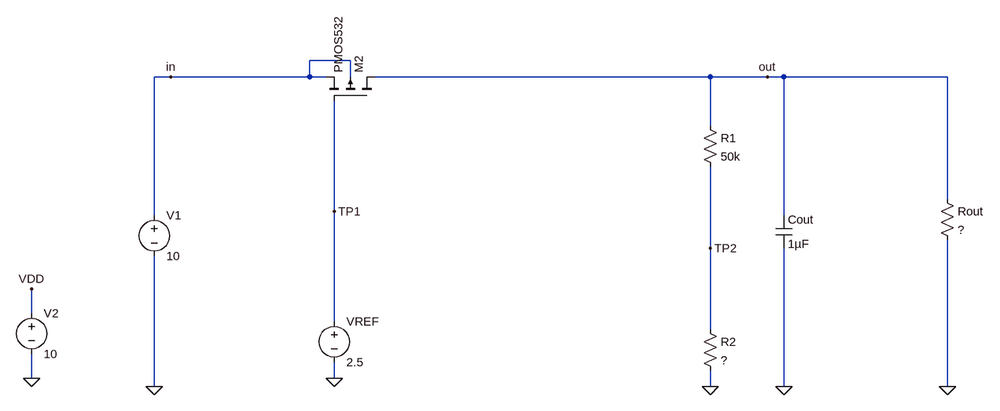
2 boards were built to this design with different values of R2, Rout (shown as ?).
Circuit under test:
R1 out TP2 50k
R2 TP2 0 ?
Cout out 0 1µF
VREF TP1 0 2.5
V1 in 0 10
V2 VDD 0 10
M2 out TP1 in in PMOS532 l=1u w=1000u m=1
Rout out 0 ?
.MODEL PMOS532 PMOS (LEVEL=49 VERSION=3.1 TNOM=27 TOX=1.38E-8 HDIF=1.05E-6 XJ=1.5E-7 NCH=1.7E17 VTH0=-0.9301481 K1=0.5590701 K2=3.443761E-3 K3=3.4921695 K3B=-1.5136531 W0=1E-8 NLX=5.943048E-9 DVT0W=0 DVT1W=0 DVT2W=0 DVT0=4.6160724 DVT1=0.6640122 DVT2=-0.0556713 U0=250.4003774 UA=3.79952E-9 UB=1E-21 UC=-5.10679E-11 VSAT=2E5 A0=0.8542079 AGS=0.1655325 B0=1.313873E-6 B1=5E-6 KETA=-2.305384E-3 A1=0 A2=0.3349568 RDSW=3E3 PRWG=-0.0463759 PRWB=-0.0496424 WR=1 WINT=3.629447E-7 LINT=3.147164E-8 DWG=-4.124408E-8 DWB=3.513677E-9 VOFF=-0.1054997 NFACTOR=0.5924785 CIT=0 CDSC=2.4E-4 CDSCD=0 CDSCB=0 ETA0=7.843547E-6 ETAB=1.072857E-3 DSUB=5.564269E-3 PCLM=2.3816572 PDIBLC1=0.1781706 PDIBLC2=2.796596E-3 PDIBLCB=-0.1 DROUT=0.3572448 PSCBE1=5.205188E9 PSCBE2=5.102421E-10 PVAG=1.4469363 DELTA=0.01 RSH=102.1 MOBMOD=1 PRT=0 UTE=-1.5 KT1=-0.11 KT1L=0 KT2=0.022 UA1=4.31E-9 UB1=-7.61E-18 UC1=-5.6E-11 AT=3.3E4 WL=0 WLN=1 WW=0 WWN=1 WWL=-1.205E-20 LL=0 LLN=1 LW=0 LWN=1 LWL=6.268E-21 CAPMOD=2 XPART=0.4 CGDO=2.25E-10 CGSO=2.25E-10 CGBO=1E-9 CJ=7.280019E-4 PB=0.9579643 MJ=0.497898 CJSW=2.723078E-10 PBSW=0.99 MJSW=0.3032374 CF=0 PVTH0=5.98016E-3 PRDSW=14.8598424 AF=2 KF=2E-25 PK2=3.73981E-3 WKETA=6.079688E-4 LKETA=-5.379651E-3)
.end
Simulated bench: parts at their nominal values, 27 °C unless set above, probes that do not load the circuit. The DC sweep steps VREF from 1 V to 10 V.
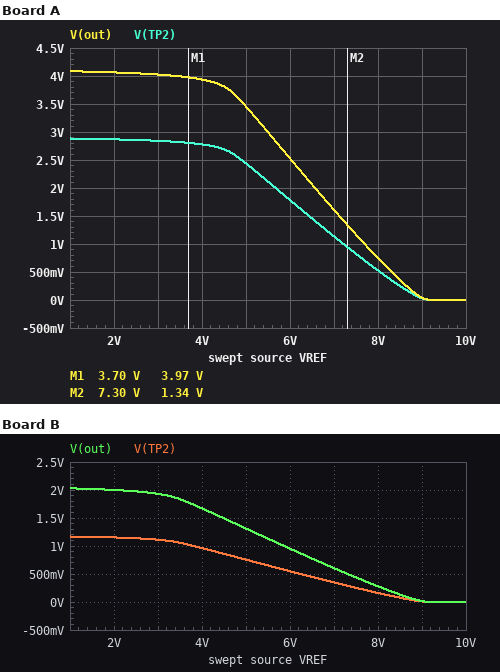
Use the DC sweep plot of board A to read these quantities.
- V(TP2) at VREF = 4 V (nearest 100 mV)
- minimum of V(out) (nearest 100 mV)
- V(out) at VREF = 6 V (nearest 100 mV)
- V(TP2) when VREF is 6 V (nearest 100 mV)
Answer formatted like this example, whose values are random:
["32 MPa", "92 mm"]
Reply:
["2.8 V", "0 V", "2.5 V", "1.8 V"]
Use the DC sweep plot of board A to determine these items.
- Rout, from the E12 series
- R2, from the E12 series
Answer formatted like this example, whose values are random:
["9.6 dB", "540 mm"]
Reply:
["150 Ω", "120 kΩ"]
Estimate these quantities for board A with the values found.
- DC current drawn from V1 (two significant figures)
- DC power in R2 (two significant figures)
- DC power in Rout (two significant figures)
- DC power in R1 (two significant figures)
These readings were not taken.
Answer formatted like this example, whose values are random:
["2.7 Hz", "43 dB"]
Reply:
["27 mA", "68 µW", "110 mW", "28 µW"]
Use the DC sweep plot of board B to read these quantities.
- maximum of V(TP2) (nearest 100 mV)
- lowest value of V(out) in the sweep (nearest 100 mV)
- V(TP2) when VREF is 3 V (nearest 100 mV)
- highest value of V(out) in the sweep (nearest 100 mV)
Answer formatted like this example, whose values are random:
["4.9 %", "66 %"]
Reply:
["1.2 V", "0 V", "1.1 V", "2.0 V"]
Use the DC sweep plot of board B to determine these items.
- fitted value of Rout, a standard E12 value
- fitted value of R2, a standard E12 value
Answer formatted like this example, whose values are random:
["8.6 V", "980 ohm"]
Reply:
["56 Ω", "68 kΩ"]
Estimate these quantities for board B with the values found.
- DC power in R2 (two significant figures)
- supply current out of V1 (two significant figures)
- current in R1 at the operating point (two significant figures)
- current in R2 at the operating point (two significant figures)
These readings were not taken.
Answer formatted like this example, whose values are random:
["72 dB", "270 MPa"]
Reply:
["19 µW", "35 mA", "17 µA", "17 µA"]
